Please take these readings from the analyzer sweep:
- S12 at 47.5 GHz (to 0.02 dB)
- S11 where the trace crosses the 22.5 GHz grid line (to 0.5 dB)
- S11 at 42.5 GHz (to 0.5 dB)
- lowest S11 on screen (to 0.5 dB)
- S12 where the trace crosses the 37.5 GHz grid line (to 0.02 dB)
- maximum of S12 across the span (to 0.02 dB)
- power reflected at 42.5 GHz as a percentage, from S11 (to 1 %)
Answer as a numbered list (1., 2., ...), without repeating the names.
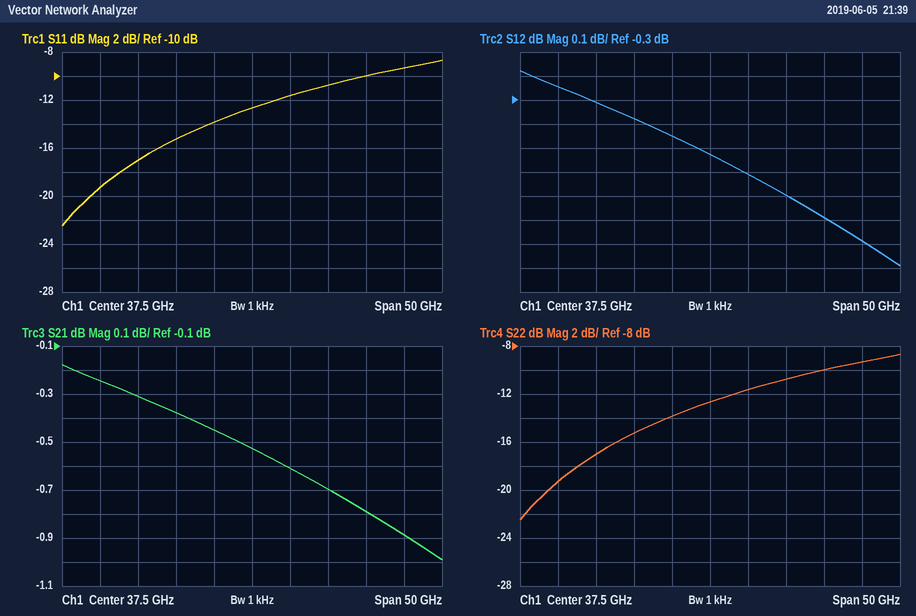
1. -0.70 dB
2. -17.0 dB
3. -11.5 dB
4. -22.5 dB
5. -0.52 dB
6. -0.18 dB
7. 7 %
